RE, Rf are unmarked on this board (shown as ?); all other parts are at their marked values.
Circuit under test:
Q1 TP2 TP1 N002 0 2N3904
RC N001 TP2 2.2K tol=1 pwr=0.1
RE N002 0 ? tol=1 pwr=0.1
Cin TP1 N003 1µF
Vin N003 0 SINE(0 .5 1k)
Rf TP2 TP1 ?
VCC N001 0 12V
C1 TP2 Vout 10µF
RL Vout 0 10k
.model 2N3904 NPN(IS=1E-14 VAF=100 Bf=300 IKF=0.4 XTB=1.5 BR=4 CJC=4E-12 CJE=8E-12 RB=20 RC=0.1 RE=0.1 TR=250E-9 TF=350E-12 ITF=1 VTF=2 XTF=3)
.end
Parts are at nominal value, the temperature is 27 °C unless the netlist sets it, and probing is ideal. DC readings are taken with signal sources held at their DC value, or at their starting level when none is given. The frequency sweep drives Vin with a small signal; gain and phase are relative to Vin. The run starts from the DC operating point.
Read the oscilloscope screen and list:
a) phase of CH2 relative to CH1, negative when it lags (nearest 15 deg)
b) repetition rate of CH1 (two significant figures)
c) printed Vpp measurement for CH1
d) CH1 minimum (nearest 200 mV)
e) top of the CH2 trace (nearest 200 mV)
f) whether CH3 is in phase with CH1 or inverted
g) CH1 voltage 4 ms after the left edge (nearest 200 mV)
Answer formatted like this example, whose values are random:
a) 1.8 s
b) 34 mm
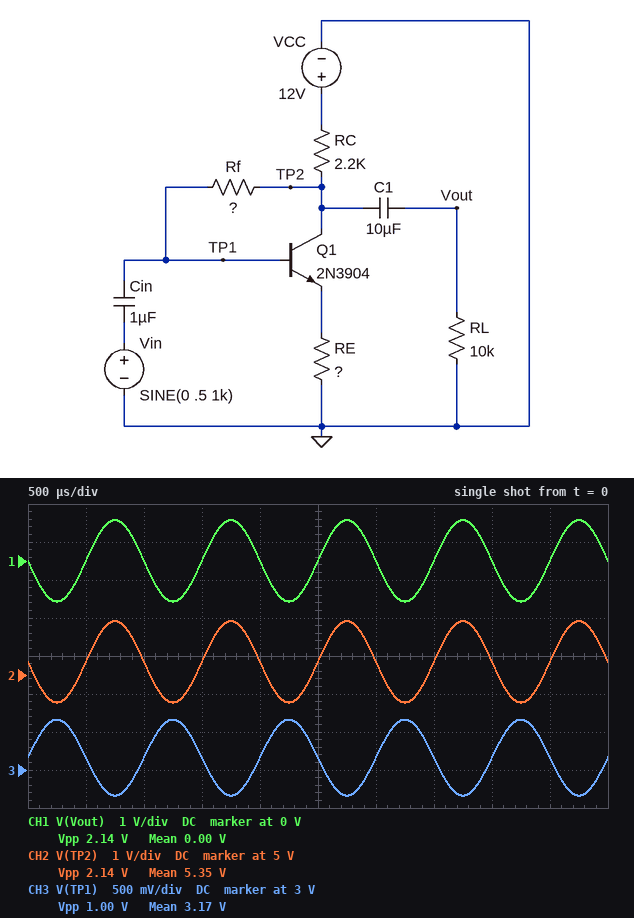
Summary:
a) 0 deg
b) 1.0 kHz
c) 2.14 V
d) -1.0 V
e) 6.4 V
f) inverted
g) 0 V
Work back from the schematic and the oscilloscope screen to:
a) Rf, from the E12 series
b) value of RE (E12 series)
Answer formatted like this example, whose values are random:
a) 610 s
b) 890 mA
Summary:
a) 220 kΩ
b) 820 Ω
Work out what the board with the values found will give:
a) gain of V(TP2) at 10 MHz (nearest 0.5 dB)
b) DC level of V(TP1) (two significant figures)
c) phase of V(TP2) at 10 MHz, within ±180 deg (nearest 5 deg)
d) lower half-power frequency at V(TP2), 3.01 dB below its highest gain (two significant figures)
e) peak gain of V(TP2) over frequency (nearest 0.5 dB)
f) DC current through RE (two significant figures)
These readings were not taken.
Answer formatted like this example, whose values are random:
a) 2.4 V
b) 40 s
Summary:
a) 6.5 dB
b) 3.2 V
c) 155 deg
d) 2.7 Hz
e) 6.5 dB
f) 3.0 mA
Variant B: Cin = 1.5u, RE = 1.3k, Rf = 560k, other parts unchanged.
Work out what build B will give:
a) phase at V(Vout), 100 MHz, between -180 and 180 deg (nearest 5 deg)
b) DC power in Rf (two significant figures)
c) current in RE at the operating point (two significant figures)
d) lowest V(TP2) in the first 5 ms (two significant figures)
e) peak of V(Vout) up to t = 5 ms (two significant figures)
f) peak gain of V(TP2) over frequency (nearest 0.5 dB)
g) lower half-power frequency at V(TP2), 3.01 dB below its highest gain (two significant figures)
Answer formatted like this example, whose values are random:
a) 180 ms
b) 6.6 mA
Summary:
a) 45 deg
b) 26 µW
c) 2.1 mA
d) 6.6 V
e) 680 mV
f) 3.0 dB
g) 580 mHz
